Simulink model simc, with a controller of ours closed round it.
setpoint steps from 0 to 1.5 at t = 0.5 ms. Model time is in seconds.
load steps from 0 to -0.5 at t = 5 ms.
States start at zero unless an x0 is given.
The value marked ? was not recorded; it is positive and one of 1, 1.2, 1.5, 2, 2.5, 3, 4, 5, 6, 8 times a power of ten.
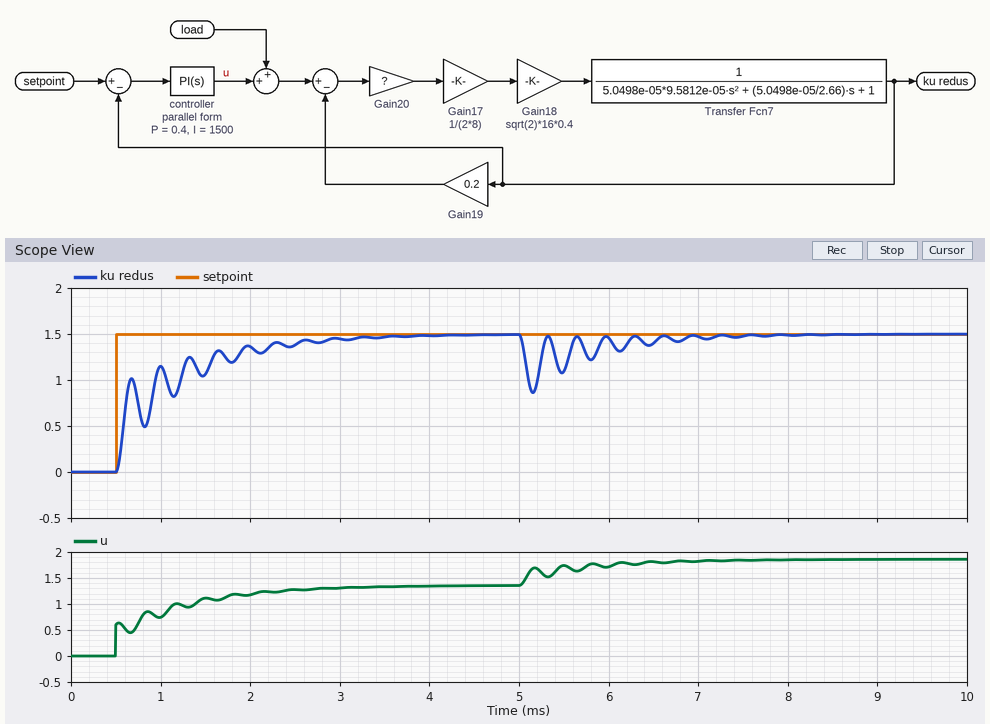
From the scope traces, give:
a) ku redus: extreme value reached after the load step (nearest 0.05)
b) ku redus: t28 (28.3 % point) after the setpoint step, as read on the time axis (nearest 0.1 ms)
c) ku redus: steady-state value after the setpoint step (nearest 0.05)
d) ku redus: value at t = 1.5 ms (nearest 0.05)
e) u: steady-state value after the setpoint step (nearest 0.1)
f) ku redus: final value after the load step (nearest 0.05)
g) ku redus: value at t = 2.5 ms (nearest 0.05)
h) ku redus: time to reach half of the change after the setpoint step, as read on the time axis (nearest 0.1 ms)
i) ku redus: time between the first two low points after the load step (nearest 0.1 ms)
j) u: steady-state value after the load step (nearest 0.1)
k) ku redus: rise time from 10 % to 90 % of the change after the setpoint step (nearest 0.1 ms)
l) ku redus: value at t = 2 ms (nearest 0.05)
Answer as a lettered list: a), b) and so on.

a) 0.85
b) 0.6 ms
c) 1.50
d) 1.05
e) 1.4
f) 1.50
g) 1.40
h) 0.6 ms
i) 0.3 ms
j) 1.9
k) 1.4 ms
l) 1.35
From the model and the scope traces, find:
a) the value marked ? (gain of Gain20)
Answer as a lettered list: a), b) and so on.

a) 2.5
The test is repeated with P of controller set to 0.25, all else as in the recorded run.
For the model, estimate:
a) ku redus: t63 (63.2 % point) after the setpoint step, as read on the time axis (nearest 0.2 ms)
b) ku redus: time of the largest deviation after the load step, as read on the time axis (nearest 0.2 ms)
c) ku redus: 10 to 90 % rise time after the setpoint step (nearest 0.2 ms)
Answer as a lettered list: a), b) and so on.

a) 1.0 ms
b) 5.2 ms
c) 1.4 ms
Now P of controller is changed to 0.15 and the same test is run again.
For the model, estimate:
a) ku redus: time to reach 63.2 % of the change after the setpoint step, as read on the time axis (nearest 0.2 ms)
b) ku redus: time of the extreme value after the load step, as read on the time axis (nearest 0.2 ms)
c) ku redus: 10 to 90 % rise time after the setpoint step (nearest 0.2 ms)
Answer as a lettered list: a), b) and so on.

a) 1.0 ms
b) 5.2 ms
c) 1.4 ms
